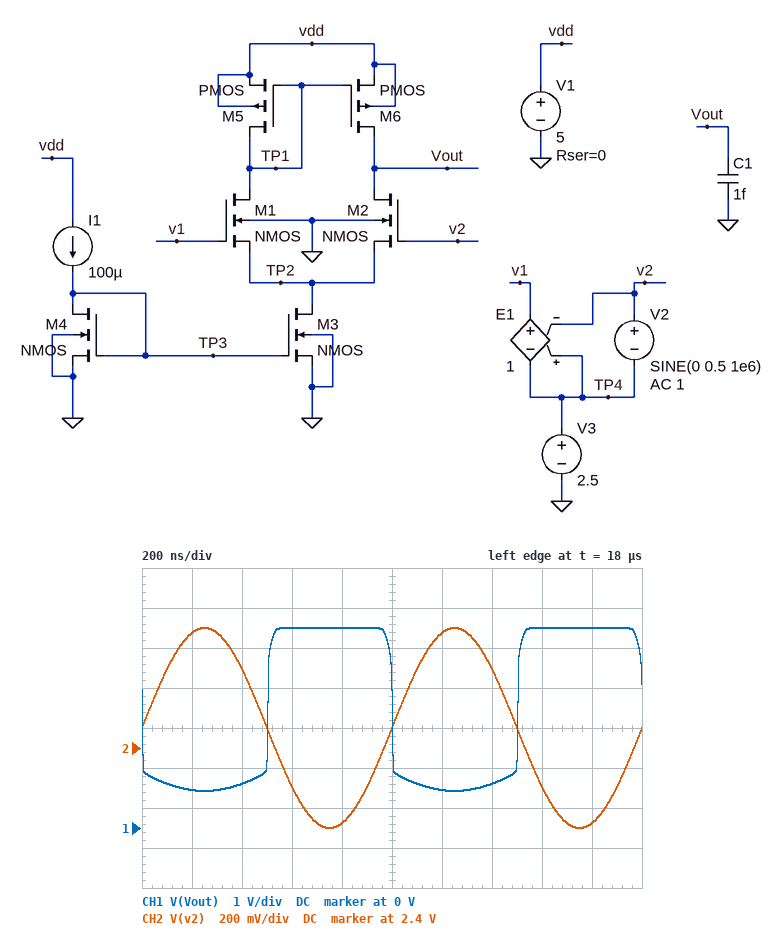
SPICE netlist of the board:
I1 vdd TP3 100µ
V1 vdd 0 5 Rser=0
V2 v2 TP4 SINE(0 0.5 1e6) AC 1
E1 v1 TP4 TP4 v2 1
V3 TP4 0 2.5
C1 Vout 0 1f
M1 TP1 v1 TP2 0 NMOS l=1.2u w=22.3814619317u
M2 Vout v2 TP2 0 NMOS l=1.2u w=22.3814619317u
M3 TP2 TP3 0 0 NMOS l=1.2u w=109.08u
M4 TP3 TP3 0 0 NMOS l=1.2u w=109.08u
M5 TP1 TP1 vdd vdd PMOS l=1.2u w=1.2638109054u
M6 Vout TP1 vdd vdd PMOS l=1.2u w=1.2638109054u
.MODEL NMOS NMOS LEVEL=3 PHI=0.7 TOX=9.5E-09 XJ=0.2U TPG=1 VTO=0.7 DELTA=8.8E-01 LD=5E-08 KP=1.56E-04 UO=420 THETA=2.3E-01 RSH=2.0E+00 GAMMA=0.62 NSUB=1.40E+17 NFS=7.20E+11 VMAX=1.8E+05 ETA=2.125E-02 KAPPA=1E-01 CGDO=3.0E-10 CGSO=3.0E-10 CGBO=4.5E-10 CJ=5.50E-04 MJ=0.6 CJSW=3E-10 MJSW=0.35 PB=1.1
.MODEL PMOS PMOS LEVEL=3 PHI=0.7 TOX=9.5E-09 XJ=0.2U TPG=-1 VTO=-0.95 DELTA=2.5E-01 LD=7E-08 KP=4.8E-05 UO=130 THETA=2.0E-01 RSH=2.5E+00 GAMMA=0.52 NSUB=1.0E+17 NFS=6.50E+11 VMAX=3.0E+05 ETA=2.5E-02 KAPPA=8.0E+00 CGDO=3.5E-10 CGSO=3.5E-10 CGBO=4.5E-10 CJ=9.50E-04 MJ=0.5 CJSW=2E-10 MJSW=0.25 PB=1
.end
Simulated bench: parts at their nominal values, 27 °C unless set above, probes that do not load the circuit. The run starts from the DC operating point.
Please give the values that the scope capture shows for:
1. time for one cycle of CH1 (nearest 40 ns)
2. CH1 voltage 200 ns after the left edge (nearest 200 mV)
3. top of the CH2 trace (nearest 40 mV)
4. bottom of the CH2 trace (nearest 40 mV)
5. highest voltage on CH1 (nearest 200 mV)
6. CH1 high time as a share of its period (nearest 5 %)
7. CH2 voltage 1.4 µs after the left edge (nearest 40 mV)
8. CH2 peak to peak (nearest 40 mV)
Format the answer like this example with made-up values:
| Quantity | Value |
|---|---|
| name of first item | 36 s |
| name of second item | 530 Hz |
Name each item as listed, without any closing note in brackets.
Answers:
| Quantity | Value |
|---|---|
| time for one cycle of CH1 | 1.00 µs |
| CH1 voltage 200 ns after the left edge | 1.0 V |
| top of the CH2 trace | 3.00 V |
| bottom of the CH2 trace | 2.00 V |
| highest voltage on CH1 | 5.0 V |
| CH1 high time as a share of its period | 50 % |
| CH2 voltage 1.4 µs after the left edge | 2.80 V |
| CH2 peak to peak | 1.00 V |
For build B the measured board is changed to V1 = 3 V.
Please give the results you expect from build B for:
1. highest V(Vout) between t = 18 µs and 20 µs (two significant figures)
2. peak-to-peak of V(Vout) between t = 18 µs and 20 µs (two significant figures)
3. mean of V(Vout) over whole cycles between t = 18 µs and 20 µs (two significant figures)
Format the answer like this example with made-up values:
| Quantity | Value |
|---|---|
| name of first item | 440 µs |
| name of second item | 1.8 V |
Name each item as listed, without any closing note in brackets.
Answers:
| Quantity | Value |
|---|---|
| highest V(Vout) between t = 18 µs and 20 µs | 450 mV |
| peak-to-peak of V(Vout) between t = 18 µs and 20 µs | 22 mV |
| mean of V(Vout) over whole cycles between t = 18 µs and 20 µs | 440 mV |
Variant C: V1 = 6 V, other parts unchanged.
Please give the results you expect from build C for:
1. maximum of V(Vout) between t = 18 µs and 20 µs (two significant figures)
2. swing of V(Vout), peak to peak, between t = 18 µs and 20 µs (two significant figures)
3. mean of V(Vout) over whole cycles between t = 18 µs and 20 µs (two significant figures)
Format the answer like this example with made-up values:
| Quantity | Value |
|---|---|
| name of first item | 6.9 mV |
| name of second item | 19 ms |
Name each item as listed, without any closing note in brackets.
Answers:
| Quantity | Value |
|---|---|
| maximum of V(Vout) between t = 18 µs and 20 µs | 6.0 V |
| swing of V(Vout), peak to peak, between t = 18 µs and 20 µs | 5.1 V |
| mean of V(Vout) over whole cycles between t = 18 µs and 20 µs | 3.5 V |
